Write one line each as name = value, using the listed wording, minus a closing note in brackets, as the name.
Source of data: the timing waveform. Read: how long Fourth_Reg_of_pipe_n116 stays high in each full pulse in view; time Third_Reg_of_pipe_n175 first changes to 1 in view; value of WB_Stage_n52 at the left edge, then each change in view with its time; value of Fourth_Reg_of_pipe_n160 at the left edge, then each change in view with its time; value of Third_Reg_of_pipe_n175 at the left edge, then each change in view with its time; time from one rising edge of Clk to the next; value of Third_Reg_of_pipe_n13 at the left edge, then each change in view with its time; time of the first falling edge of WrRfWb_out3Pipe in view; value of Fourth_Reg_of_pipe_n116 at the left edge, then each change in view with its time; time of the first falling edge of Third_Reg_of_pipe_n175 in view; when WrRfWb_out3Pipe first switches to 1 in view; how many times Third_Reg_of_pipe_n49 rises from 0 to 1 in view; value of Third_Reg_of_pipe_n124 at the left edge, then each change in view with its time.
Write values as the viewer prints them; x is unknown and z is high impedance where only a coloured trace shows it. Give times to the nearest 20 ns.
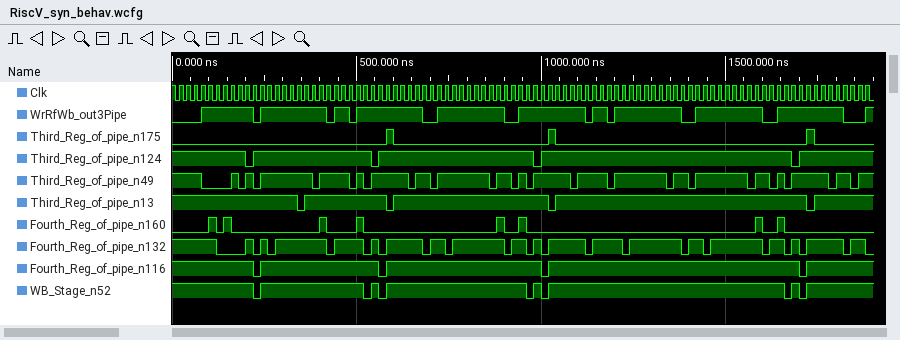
how long Fourth_Reg_of_pipe_n116 stays high in each full pulse in view = 320 ns, 420 ns, 680 ns
time Third_Reg_of_pipe_n175 first changes to 1 in view = 580 ns
value of WB_Stage_n52 at the left edge, then each change in view with its time = 1, 0 at 220 ns, 1 at 240 ns, 0 at 520 ns, 1 at 540 ns, 0 at 560 ns, 1 at 580 ns, 0 at 960 ns, 1 at 980 ns, 0 at 1000 ns, 1 at 1020 ns, 0 at 1660 ns, 1 at 1680 ns, 0 at 1700 ns, 1 at 1720 ns
value of Fourth_Reg_of_pipe_n160 at the left edge, then each change in view with its time = 0, 1 at 100 ns, 0 at 120 ns, 1 at 140 ns, 0 at 160 ns, 1 at 400 ns, 0 at 420 ns, 1 at 500 ns, 0 at 520 ns, 1 at 880 ns, 0 at 900 ns, 1 at 940 ns, 0 at 960 ns, 1 at 1580 ns, 0 at 1600 ns, 1 at 1640 ns, 0 at 1660 ns
value of Third_Reg_of_pipe_n175 at the left edge, then each change in view with its time = 0, 1 at 580 ns, 0 at 600 ns, 1 at 1020 ns, 0 at 1040 ns, 1 at 1720 ns, 0 at 1740 ns
time from one rising edge of Clk to the next = 20 ns
value of Third_Reg_of_pipe_n13 at the left edge, then each change in view with its time = 1, 0 at 340 ns, 1 at 360 ns, 0 at 580 ns, 1 at 600 ns, 0 at 1020 ns, 1 at 1040 ns, 0 at 1720 ns, 1 at 1740 ns
time of the first falling edge of WrRfWb_out3Pipe in view = 220 ns
value of Fourth_Reg_of_pipe_n116 at the left edge, then each change in view with its time = 1, 0 at 220 ns, 1 at 240 ns, 0 at 560 ns, 1 at 580 ns, 0 at 1000 ns, 1 at 1020 ns, 0 at 1700 ns, 1 at 1720 ns
time of the first falling edge of Third_Reg_of_pipe_n175 in view = 600 ns
when WrRfWb_out3Pipe first switches to 1 in view = 80 ns
how many times Third_Reg_of_pipe_n49 rises from 0 to 1 in view = 20
value of Third_Reg_of_pipe_n124 at the left edge, then each change in view with its time = 1, 0 at 200 ns, 1 at 220 ns, 0 at 540 ns, 1 at 560 ns, 0 at 980 ns, 1 at 1000 ns, 0 at 1680 ns, 1 at 1700 ns
